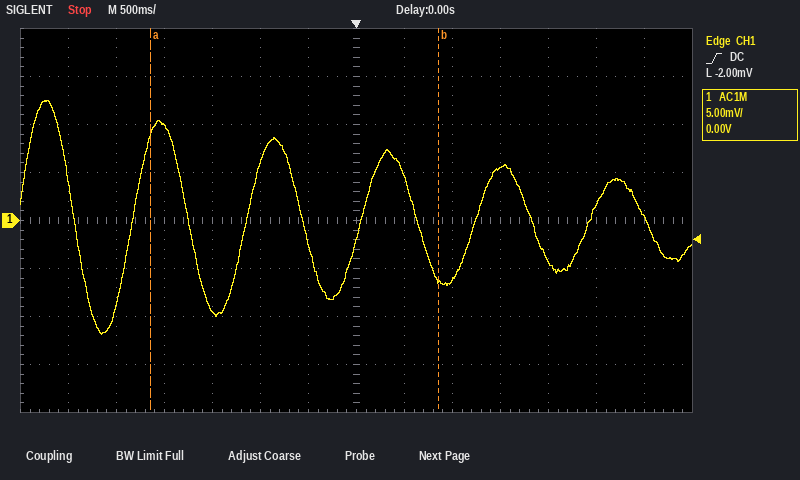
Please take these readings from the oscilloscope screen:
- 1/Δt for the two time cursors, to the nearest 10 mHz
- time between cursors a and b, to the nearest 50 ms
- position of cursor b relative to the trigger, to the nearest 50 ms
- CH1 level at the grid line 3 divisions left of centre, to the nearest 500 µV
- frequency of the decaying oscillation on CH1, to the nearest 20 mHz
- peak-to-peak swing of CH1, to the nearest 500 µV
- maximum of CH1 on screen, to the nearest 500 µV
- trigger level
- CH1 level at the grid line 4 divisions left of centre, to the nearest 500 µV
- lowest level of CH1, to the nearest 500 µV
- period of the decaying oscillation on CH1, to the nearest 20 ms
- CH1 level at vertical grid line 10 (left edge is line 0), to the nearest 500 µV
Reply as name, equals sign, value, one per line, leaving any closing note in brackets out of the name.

1/Δt for the two time cursors, to the nearest 10 mHz = 330 mHz
time between cursors a and b, to the nearest 50 ms = 3.00 s
position of cursor b relative to the trigger, to the nearest 50 ms = +850 ms
CH1 level at the grid line 3 divisions left of centre, to the nearest 500 µV = -9.5 mV
frequency of the decaying oscillation on CH1, to the nearest 20 mHz = 840 mHz
peak-to-peak swing of CH1, to the nearest 500 µV = 24.5 mV
maximum of CH1 on screen, to the nearest 500 µV = 12.5 mV
trigger level = -2.00 mV
CH1 level at the grid line 4 divisions left of centre, to the nearest 500 µV = 10.0 mV
lowest level of CH1, to the nearest 500 µV = -12.0 mV
period of the decaying oscillation on CH1, to the nearest 20 ms = 1.18 s
CH1 level at vertical grid line 10 (left edge is line 0), to the nearest 500 µV = 5.5 mV
